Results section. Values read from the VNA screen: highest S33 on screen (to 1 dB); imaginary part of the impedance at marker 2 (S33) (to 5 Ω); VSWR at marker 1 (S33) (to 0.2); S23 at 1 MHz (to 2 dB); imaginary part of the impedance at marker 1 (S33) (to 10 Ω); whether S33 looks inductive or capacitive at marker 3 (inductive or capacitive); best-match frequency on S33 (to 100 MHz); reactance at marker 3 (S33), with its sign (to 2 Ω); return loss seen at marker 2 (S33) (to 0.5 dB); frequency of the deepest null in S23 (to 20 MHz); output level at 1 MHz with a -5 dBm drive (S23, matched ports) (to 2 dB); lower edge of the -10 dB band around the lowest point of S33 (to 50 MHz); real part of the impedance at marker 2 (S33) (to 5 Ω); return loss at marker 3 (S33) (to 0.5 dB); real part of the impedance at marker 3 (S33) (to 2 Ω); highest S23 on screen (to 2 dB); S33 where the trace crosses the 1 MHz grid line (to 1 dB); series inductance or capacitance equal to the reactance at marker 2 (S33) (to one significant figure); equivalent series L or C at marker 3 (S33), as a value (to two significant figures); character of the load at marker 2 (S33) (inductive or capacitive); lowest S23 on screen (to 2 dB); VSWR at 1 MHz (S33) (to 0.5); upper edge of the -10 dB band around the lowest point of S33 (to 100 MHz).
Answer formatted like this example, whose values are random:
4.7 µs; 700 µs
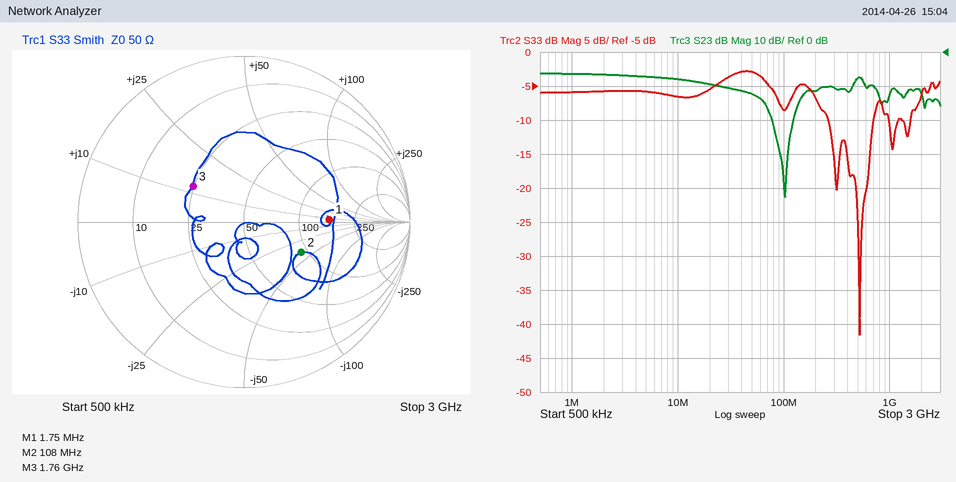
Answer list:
-3 dB; -40 Ω; 3.2; -6 dB; +10 Ω; inductive; 500 MHz; +12 Ω; 8.0 dB; 100 MHz; -12 dBm; 250 MHz; 90 Ω; 8.5 dB; 24 Ω; -6 dB; -6 dB; 40 pF; 1.1 nH; capacitive; -42 dB; 3.0; 700 MHz
